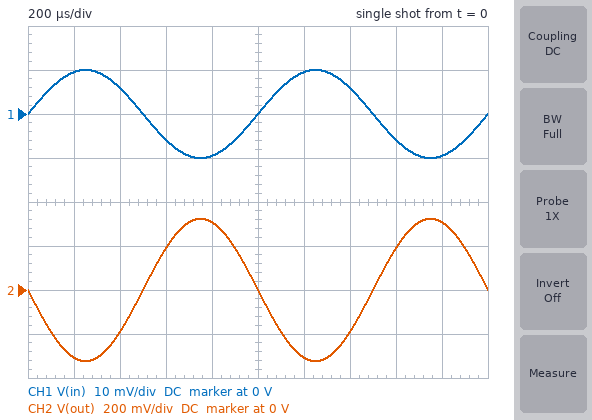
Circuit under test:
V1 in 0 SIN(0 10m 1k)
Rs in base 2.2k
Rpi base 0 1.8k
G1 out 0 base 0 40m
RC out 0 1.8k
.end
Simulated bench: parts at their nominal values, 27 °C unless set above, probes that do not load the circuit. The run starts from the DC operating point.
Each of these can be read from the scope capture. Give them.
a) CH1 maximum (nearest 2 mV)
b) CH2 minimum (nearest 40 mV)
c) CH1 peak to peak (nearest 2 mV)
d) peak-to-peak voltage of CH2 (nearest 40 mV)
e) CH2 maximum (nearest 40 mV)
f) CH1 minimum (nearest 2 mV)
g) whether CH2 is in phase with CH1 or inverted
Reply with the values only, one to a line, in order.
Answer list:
10 mV
-320 mV
20 mV
640 mV
320 mV
-10 mV
inverted
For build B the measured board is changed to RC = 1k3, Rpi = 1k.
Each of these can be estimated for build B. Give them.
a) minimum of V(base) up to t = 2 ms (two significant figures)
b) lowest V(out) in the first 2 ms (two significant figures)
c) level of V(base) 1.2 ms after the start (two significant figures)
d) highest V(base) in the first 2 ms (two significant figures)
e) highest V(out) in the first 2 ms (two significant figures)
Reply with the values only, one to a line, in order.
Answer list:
-3.1 mV
-160 mV
3.0 mV
3.1 mV
160 mV
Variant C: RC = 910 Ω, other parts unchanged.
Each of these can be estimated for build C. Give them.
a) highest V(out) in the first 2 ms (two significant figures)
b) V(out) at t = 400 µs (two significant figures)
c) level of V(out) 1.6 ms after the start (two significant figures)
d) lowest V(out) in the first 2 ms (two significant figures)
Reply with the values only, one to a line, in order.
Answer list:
160 mV
-96 mV
96 mV
-160 mV
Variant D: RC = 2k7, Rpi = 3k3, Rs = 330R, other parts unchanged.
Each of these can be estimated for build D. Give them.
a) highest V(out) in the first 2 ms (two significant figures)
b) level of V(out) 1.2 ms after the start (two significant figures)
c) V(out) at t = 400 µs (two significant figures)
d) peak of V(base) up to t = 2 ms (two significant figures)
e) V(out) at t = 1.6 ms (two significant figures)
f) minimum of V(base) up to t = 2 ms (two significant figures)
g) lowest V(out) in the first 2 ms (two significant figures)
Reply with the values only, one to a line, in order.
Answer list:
980 mV
-930 mV
-580 mV
9.1 mV
580 mV
-9.1 mV
-980 mV
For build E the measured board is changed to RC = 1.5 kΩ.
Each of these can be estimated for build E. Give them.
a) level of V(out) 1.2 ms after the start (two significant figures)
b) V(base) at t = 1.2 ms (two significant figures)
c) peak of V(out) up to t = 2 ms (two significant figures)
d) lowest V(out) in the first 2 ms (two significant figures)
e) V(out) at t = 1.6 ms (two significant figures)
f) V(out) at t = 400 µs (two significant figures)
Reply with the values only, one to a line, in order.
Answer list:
-260 mV
4.3 mV
270 mV
-270 mV
160 mV
-160 mV
